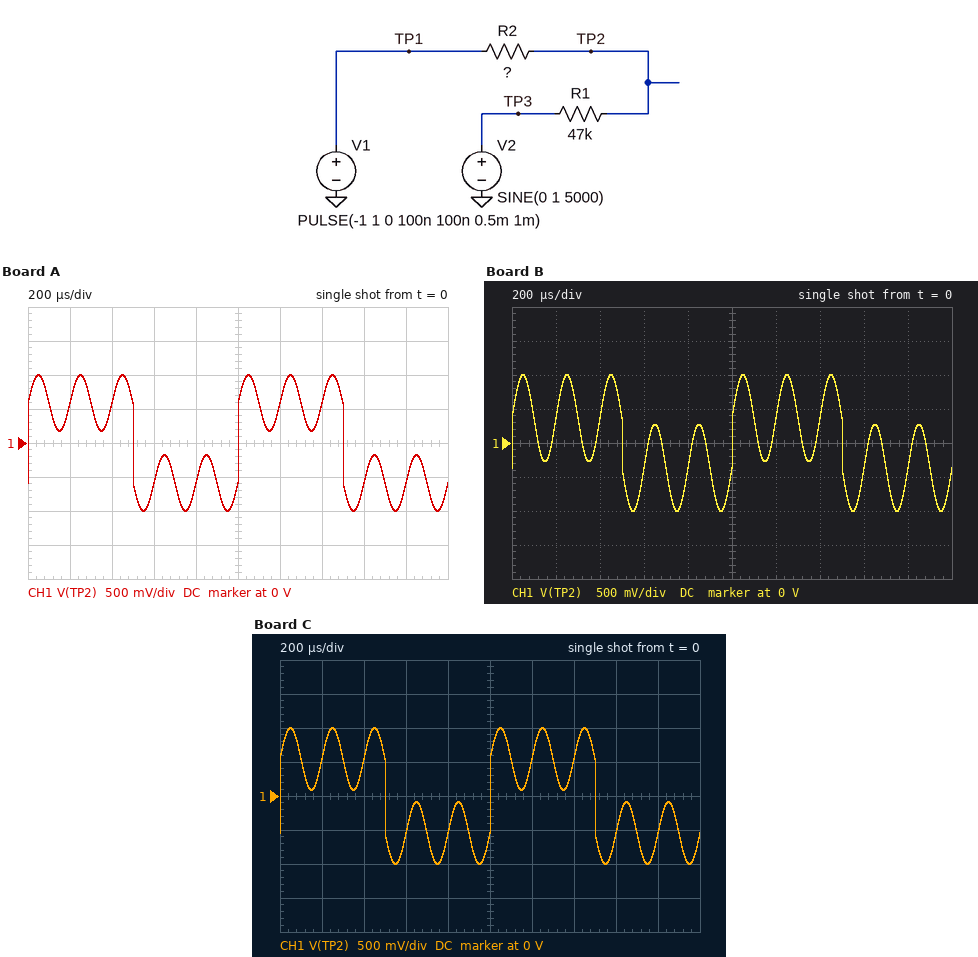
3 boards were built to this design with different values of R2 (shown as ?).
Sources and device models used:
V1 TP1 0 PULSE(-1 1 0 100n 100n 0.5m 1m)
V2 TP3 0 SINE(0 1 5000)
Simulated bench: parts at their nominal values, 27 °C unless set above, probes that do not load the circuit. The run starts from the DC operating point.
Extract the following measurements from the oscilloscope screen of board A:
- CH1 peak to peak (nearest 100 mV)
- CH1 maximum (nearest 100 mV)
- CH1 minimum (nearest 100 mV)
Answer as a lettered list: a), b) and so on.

a) 2.0 V
b) 1.0 V
c) -1.0 V
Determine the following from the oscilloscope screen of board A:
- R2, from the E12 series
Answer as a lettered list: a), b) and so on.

a) 33 kΩ
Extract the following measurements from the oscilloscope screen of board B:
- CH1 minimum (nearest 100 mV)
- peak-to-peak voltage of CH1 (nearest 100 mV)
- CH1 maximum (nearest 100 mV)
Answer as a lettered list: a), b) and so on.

a) -1.0 V
b) 2.0 V
c) 1.0 V
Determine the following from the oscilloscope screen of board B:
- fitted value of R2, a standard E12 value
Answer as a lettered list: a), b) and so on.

a) 82 kΩ
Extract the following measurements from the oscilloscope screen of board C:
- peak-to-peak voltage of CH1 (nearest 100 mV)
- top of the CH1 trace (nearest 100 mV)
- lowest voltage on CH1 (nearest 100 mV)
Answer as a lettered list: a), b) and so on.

a) 2.0 V
b) 1.0 V
c) -1.0 V
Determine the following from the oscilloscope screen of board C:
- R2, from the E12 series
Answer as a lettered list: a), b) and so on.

a) 39 kΩ
